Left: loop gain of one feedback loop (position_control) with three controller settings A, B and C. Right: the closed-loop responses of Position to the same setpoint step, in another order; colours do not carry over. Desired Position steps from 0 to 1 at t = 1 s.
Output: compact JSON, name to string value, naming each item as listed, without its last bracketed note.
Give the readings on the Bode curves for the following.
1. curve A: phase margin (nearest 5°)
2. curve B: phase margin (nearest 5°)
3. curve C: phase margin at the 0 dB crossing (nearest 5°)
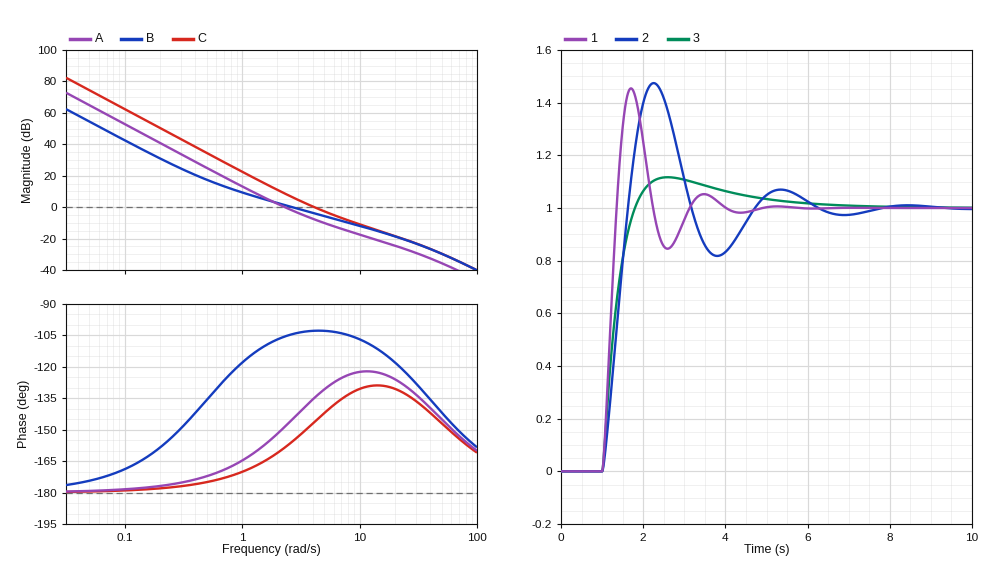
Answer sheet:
{"curve A: phase margin": "30°", "curve B: phase margin": "75°", "curve C: phase margin at the 0 dB crossing": "35°"}
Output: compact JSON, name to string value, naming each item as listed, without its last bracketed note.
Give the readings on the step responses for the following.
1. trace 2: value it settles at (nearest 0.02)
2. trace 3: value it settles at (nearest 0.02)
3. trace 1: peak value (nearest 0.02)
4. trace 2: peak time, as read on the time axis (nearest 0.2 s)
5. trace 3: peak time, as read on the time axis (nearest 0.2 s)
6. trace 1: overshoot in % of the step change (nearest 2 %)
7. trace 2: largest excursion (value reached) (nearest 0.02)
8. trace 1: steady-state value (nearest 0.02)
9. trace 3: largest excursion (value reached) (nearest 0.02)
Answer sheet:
{"trace 2: value it settles at": "1.00", "trace 3: value it settles at": "1.00", "trace 1: peak value": "1.46", "trace 2: peak time, as read on the time axis": "2.2 s", "trace 3: peak time, as read on the time axis": "2.6 s", "trace 1: overshoot in % of the step change": "46 %", "trace 2: largest excursion (value reached)": "1.48", "trace 1: steady-state value": "1.00", "trace 3: largest excursion (value reached)": "1.12"}
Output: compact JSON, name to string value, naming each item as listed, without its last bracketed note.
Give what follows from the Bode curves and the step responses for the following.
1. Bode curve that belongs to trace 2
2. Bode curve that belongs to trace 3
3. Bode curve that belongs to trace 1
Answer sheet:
{"Bode curve that belongs to trace 2": "A", "Bode curve that belongs to trace 3": "B", "Bode curve that belongs to trace 1": "C"}
